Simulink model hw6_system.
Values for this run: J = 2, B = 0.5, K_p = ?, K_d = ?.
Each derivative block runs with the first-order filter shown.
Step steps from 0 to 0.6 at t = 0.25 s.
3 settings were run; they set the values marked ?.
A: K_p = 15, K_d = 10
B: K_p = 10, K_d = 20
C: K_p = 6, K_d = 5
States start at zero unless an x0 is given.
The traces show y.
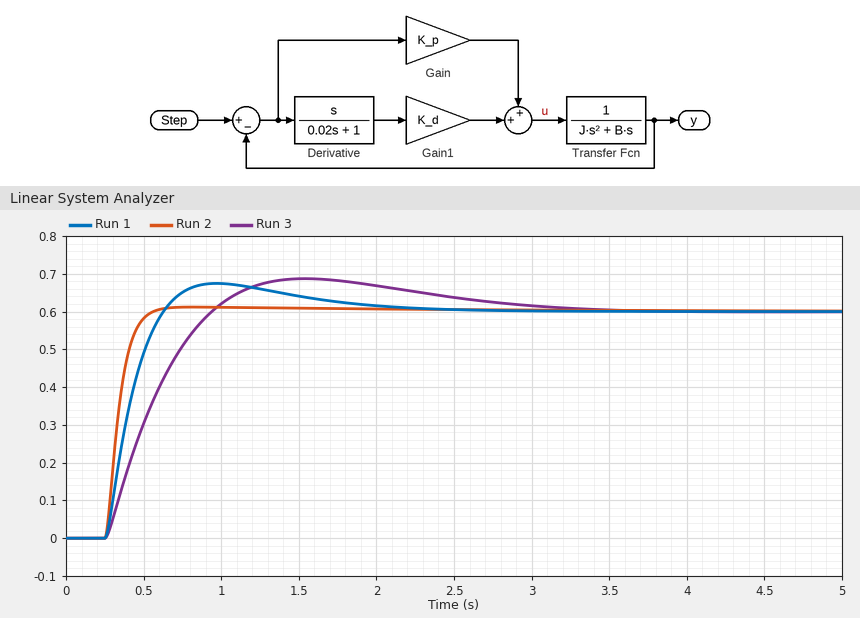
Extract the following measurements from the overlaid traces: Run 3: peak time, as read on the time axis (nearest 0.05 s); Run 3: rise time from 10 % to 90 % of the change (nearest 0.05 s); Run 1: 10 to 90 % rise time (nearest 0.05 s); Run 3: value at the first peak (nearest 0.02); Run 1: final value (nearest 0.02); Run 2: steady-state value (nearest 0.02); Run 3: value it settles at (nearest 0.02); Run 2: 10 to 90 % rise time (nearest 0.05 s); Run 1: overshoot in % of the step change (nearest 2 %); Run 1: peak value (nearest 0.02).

1.55 s
0.50 s
0.25 s
0.68
0.60
0.60
0.60
0.15 s
12 %
0.68
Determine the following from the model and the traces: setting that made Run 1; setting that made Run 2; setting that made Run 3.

A
B
C
